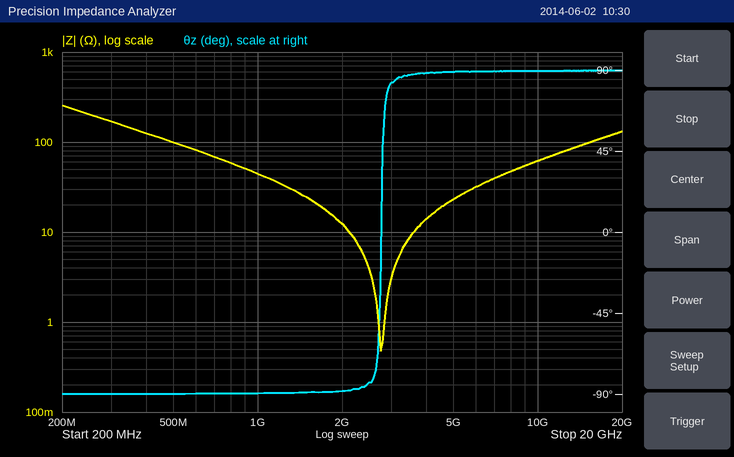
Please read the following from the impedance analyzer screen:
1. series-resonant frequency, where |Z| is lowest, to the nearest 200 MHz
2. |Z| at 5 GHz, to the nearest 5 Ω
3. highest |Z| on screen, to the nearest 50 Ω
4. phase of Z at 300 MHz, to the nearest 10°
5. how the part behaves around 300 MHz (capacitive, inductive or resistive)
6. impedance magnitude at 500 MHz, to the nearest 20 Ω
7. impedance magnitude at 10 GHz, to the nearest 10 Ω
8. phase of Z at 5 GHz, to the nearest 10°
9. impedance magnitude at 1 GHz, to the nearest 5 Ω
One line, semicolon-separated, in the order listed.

2.8 GHz; 25 Ω; 250 Ω; -90°; capacitive; 100 Ω; 60 Ω; 90°; 45 Ω
